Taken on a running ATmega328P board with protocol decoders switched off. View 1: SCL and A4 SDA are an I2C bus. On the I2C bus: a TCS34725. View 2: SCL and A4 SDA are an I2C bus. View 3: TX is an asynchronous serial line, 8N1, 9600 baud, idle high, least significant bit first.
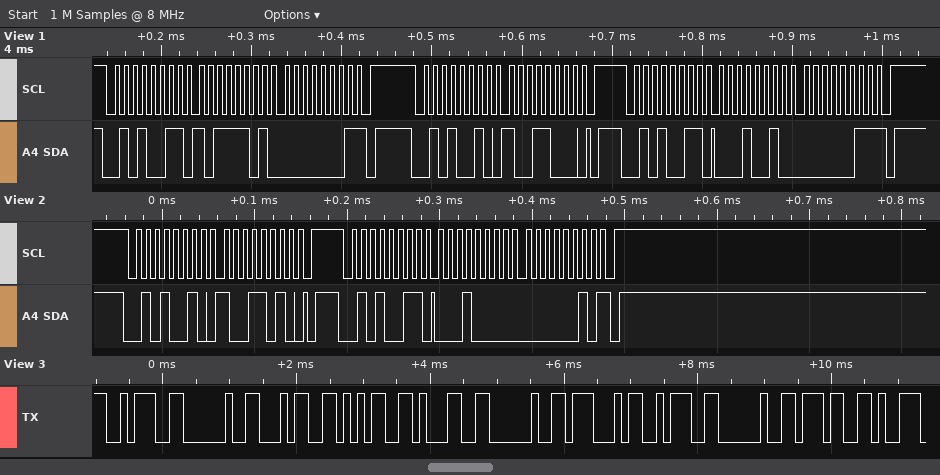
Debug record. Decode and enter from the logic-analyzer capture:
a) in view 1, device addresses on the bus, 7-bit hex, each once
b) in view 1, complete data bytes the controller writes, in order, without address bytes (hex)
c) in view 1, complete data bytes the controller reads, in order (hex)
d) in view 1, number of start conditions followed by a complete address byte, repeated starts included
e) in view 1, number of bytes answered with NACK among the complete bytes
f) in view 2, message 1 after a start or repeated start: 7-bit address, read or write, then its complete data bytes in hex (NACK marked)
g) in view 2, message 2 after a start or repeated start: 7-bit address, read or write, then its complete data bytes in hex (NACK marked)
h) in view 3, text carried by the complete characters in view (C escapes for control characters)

0x29
98
BD 01 12 03
3
2
0x29 write: 9A
0x29 read: 10 02 NACK
": 451 G: 7"
